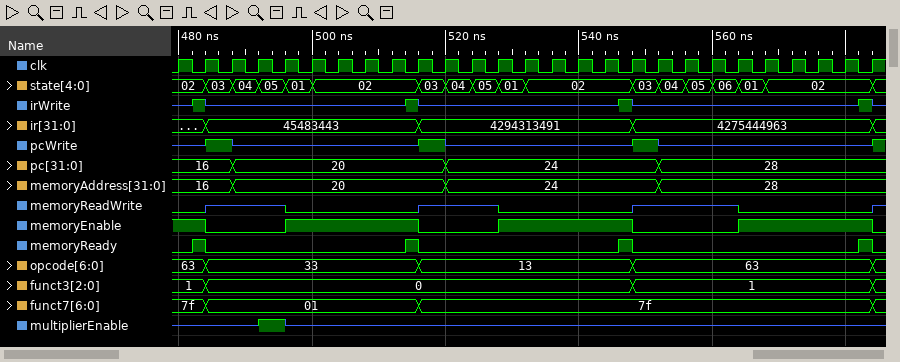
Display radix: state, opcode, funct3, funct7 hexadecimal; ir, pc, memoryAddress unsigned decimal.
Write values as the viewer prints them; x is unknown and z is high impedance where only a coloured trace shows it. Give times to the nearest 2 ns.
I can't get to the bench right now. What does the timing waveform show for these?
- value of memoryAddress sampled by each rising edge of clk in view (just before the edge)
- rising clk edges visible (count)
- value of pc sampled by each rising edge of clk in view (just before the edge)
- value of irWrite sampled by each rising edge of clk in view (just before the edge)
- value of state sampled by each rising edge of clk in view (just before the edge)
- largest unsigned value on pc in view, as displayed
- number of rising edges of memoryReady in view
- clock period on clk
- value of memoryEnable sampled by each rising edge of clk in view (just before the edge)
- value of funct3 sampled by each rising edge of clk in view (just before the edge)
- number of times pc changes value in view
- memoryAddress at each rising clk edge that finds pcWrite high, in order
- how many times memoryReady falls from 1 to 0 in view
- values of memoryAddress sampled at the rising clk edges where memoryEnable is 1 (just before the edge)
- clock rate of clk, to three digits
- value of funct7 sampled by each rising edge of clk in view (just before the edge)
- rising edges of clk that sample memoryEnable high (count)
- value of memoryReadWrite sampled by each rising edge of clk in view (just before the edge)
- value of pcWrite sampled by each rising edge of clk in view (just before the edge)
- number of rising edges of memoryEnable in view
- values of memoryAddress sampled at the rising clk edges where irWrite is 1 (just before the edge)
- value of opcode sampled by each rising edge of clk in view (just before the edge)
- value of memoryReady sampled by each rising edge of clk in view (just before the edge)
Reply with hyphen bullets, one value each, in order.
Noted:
- 16, 16, 16, 20, 20, 20, 20, 20, 20, 20, 20, 24, 24, 24, 24, 24, 24, 24, 24, 28, 28, 28, 28, 28, 28, 28, 28
- 27
- 16, 16, 16, 20, 20, 20, 20, 20, 20, 20, 20, 24, 24, 24, 24, 24, 24, 24, 24, 28, 28, 28, 28, 28, 28, 28, 28
- z 1 z z z z z z z 1 z z z z z z z 1 z z z z z z z z 1
- 02, 02, 03, 04, 05, 01, 02, 02, 02, 02, 03, 04, 05, 01, 02, 02, 02, 02, 03, 04, 05, 06, 01, 02, 02, 02, 02
- 28
- 4
- 4 ns
- 1 1 0 0 0 1 1 1 1 1 0 0 0 1 1 1 1 1 0 0 0 0 1 1 1 1 1
- 1, 1, 0, 0, 0, 0, 0, 0, 0, 0, 0, 0, 0, 0, 0, 0, 0, 0, 1, 1, 1, 1, 1, 1, 1, 1, 1
- 3
- 16, 20, 24
- 4
- 16, 16, 20, 20, 20, 20, 20, 24, 24, 24, 24, 24, 28, 28, 28, 28, 28
- 250 MHz
- 7f, 7f, 01, 01, 01, 01, 01, 01, 01, 01, 7f, 7f, 7f, 7f, 7f, 7f, 7f, 7f, 7f, 7f, 7f, 7f, 7f, 7f, 7f, 7f, 7f
- 17
- 0 0 z z z 0 0 0 0 0 z z z 0 0 0 0 0 z z z z 0 0 0 0 0
- z z 1 z z z z z z z 1 z z z z z z z 1 z z z z z z z z
- 3
- 16, 20, 24, 28
- 63, 63, 33, 33, 33, 33, 33, 33, 33, 33, 13, 13, 13, 13, 13, 13, 13, 13, 63, 63, 63, 63, 63, 63, 63, 63, 63
- 0 1 0 0 0 0 0 0 0 1 0 0 0 0 0 0 0 1 0 0 0 0 0 0 0 0 1
